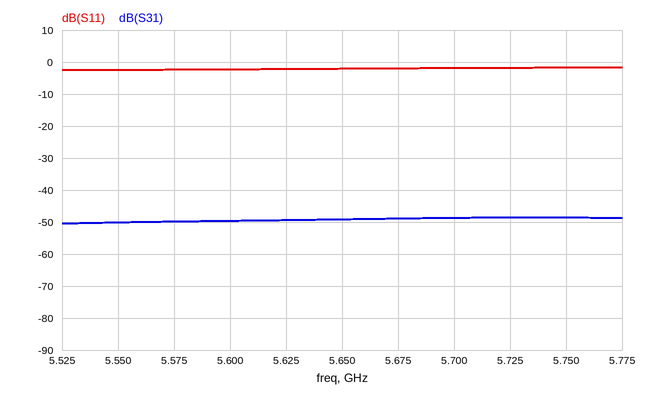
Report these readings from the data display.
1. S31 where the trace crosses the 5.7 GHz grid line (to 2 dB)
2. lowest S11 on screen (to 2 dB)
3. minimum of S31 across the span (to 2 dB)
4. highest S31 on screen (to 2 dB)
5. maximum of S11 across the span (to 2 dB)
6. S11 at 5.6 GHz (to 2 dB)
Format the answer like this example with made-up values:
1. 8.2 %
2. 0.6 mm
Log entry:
1. -48 dB
2. -2 dB
3. -50 dB
4. -48 dB
5. -2 dB
6. -2 dB
